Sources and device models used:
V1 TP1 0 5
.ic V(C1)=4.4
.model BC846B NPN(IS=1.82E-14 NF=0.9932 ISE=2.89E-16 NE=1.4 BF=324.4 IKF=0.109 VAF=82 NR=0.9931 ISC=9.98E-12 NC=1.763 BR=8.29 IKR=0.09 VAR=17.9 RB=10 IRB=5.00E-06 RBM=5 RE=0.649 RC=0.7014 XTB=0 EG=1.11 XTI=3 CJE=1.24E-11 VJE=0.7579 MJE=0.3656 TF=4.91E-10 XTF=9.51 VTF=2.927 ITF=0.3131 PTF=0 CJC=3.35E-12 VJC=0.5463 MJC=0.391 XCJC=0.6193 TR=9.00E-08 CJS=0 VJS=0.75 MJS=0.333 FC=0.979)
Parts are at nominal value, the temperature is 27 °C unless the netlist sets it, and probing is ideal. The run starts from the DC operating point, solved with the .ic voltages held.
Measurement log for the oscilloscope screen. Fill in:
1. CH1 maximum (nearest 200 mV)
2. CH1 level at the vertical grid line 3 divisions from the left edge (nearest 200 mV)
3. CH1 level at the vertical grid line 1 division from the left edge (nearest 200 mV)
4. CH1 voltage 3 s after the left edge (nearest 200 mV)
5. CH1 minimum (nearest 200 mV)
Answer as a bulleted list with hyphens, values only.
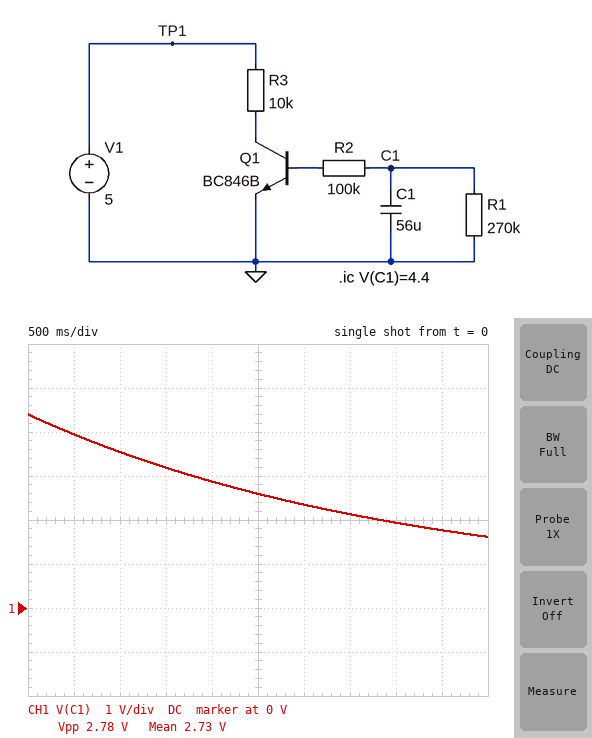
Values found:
- 4.4 V
- 3.2 V
- 4.0 V
- 2.4 V
- 1.6 V
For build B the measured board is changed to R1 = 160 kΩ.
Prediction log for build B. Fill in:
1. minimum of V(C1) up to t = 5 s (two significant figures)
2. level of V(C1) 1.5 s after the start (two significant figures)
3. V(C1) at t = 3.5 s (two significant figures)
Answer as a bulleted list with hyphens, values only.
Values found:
- 1.3 V
- 3.0 V
- 1.8 V
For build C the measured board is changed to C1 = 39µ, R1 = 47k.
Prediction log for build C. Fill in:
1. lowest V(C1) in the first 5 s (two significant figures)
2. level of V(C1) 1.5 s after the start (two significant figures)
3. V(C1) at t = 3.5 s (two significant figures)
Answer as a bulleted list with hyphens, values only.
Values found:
- 190 mV
- 1.5 V
- 440 mV
